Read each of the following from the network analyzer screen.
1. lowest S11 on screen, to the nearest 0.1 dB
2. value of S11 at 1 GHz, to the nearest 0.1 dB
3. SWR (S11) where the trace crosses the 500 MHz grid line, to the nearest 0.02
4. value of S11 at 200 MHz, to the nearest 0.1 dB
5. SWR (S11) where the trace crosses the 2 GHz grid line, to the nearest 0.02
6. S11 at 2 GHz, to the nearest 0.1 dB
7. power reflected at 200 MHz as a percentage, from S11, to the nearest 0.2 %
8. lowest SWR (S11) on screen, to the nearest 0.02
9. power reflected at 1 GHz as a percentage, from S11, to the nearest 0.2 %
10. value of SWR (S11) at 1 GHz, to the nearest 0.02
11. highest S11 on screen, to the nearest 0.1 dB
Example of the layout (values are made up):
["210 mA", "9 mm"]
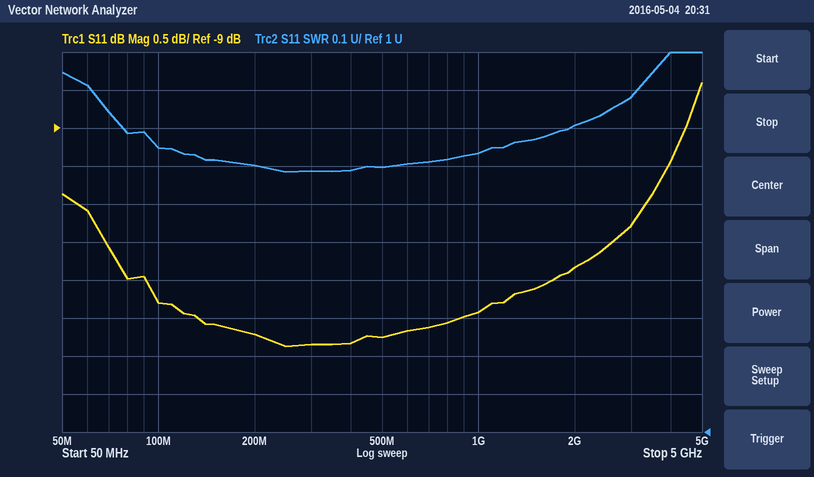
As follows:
["-11.9 dB", "-11.4 dB", "1.70", "-11.7 dB", "1.80", "-10.8 dB", "6.8 %", "1.68", "7.2 %", "1.74", "-8.4 dB"]
